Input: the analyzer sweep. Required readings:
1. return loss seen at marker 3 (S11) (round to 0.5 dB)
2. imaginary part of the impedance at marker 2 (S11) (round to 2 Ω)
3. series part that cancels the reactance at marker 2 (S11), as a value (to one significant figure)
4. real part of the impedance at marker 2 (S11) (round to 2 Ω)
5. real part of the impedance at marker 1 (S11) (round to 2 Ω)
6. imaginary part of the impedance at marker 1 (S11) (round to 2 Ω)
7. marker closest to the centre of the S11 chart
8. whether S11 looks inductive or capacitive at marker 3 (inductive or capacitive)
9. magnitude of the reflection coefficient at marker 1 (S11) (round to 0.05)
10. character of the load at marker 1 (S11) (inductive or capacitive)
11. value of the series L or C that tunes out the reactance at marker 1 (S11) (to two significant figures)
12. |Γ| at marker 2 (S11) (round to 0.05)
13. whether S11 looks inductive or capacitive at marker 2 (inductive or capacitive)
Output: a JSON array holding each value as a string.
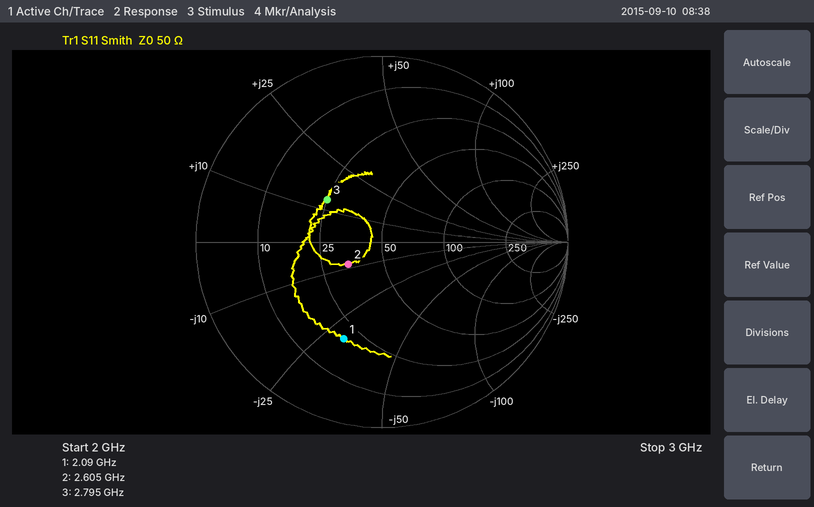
["8.5 dB", "-8 Ω", "500 pH", "34 Ω", "20 Ω", "-30 Ω", "marker 2", "inductive", "0.55", "capacitive", "2.3 nH", "0.20", "capacitive"]
